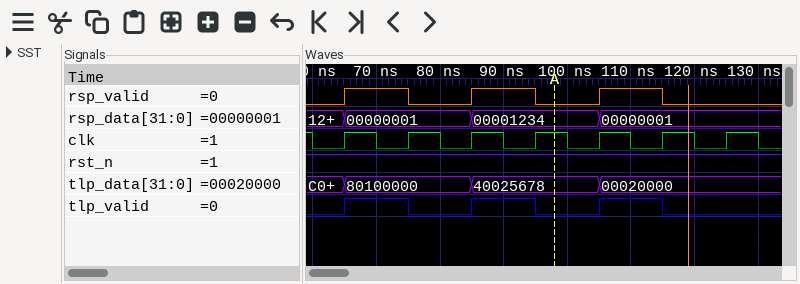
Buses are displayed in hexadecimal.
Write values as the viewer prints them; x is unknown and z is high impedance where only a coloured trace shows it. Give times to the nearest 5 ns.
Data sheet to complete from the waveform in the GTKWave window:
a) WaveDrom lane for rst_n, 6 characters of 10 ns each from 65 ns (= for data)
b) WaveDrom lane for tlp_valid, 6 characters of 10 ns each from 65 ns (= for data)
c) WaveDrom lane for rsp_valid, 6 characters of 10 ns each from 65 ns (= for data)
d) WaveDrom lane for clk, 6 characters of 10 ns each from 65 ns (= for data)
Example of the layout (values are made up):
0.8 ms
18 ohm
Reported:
{name: 'rst_n', wave: '1.....'}
{name: 'tlp_valid', wave: '101010'}
{name: 'rsp_valid', wave: '101010'}
{name: 'clk', wave: 'p.....'}
